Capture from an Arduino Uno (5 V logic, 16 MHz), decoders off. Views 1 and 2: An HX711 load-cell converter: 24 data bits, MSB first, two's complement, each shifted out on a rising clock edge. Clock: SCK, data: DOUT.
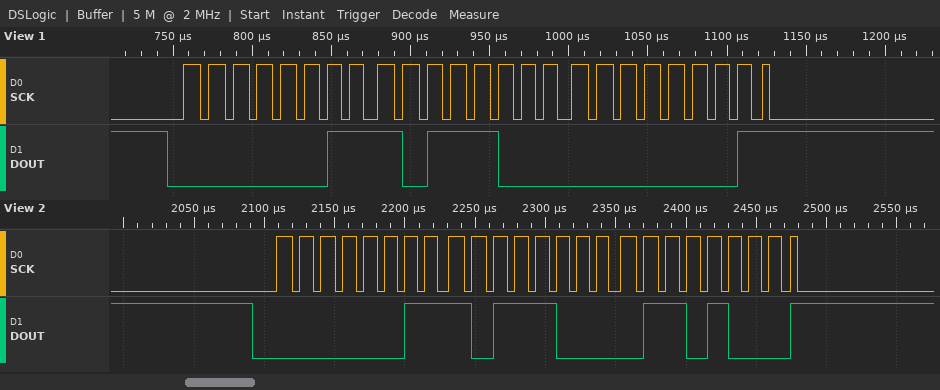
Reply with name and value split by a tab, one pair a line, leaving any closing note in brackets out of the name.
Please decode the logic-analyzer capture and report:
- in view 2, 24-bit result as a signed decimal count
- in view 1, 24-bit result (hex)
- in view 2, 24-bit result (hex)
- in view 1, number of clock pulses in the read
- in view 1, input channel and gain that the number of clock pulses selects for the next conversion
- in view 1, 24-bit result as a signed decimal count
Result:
in view 2, 24-bit result as a signed decimal count	243816
in view 1, 24-bit result	0x03B801
in view 2, 24-bit result	0x03B868
in view 1, number of clock pulses in the read	25
in view 1, input channel and gain that the number of clock pulses selects for the next conversion	channel A, gain 128
in view 1, 24-bit result as a signed decimal count	243713
